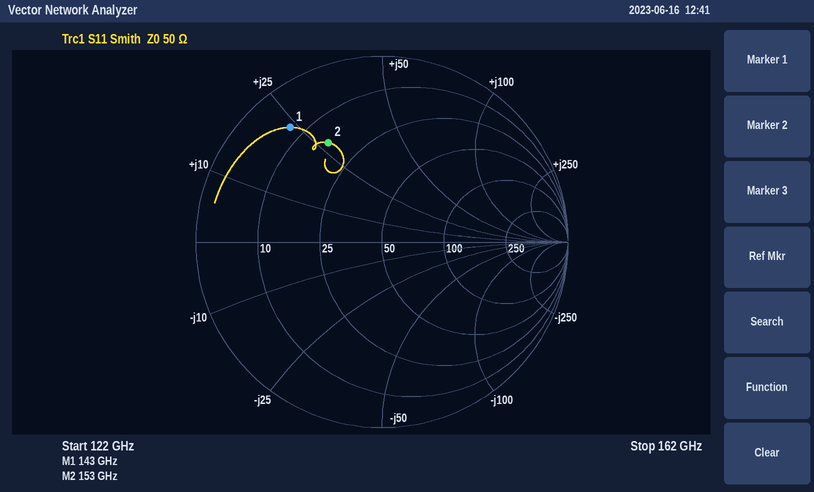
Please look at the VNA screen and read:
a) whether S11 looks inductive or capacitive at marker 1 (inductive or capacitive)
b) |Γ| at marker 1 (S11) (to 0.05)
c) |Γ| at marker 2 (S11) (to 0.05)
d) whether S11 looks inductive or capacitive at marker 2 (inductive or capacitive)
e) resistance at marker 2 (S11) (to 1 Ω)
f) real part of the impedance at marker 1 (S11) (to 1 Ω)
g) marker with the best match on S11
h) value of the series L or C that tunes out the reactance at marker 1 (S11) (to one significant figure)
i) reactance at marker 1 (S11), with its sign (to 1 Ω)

inductive
0.80
0.60
inductive
16 Ω
7 Ω
marker 2
50 fF
+24 Ω
